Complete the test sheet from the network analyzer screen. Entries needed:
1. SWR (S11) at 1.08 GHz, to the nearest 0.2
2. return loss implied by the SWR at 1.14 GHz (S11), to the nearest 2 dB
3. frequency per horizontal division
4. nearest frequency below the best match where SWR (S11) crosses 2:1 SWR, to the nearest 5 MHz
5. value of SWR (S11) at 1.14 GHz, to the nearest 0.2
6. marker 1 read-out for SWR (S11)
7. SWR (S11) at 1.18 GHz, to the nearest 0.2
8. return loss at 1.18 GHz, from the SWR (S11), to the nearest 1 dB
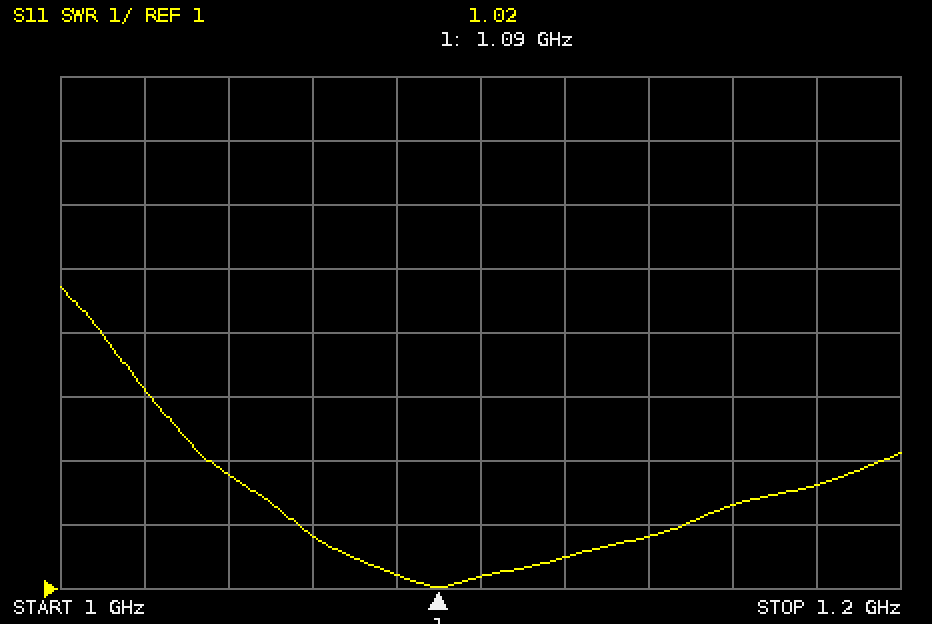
1.2
10 dB
20 MHz
1.055 GHz
1.8
1.02
2.6
7 dB
